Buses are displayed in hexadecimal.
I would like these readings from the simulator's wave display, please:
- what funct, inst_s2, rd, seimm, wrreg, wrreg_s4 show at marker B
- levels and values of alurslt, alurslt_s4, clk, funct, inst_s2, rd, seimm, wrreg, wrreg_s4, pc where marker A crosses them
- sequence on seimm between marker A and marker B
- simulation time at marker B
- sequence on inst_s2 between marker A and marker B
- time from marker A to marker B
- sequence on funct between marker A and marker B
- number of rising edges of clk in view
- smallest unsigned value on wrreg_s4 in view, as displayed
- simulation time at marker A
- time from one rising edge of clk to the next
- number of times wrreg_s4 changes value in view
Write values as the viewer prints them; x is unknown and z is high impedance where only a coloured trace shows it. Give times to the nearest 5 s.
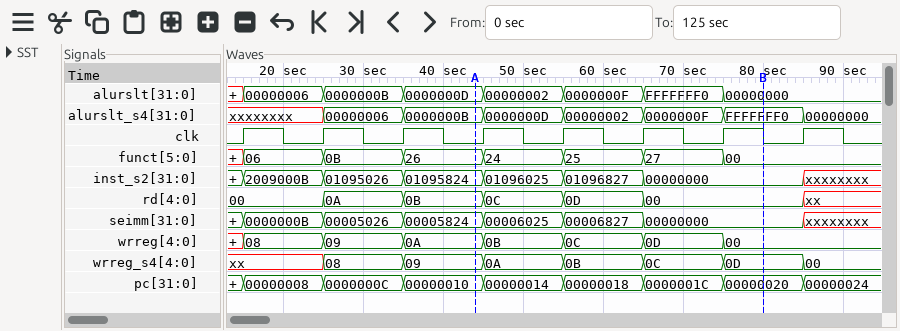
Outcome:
funct=00, inst_s2=00000000, rd=00, seimm=00000000, wrreg=00, wrreg_s4=0D
alurslt=0000000D, alurslt_s4=0000000B, clk=0, funct=26, inst_s2=01095824, rd=0B, seimm=00005824, wrreg=0A, wrreg_s4=09, pc=00000010
00005824, 00006025, 00006827, 00000000
80 s
01095824, 01096025, 01096827, 00000000
35 s
26, 24, 25, 27, 00
8
00
45 s
10 s
7
